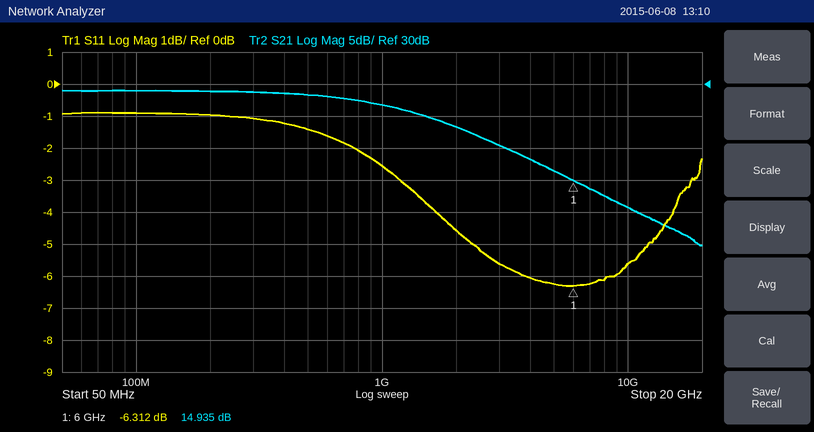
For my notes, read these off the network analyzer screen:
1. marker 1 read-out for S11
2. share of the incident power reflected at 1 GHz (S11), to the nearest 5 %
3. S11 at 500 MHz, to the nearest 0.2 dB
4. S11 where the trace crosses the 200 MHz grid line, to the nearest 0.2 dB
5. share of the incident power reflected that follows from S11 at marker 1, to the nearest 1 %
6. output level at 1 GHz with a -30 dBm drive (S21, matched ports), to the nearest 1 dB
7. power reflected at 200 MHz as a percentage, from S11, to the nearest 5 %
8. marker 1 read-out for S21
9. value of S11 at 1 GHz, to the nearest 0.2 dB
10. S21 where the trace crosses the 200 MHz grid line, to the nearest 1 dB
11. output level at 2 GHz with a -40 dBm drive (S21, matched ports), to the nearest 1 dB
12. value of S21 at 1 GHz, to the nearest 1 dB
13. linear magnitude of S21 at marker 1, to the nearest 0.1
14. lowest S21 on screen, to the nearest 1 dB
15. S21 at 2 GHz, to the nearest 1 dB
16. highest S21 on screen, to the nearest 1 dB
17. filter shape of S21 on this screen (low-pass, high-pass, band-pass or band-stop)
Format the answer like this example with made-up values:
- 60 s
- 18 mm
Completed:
- -6.312 dB
- 55 %
- -1.4 dB
- -1.0 dB
- 23 %
- -3 dBm
- 80 %
- 14.935 dB
- -2.6 dB
- 29 dB
- -17 dBm
- 27 dB
- 5.6
- 5 dB
- 23 dB
- 29 dB
- low-pass
